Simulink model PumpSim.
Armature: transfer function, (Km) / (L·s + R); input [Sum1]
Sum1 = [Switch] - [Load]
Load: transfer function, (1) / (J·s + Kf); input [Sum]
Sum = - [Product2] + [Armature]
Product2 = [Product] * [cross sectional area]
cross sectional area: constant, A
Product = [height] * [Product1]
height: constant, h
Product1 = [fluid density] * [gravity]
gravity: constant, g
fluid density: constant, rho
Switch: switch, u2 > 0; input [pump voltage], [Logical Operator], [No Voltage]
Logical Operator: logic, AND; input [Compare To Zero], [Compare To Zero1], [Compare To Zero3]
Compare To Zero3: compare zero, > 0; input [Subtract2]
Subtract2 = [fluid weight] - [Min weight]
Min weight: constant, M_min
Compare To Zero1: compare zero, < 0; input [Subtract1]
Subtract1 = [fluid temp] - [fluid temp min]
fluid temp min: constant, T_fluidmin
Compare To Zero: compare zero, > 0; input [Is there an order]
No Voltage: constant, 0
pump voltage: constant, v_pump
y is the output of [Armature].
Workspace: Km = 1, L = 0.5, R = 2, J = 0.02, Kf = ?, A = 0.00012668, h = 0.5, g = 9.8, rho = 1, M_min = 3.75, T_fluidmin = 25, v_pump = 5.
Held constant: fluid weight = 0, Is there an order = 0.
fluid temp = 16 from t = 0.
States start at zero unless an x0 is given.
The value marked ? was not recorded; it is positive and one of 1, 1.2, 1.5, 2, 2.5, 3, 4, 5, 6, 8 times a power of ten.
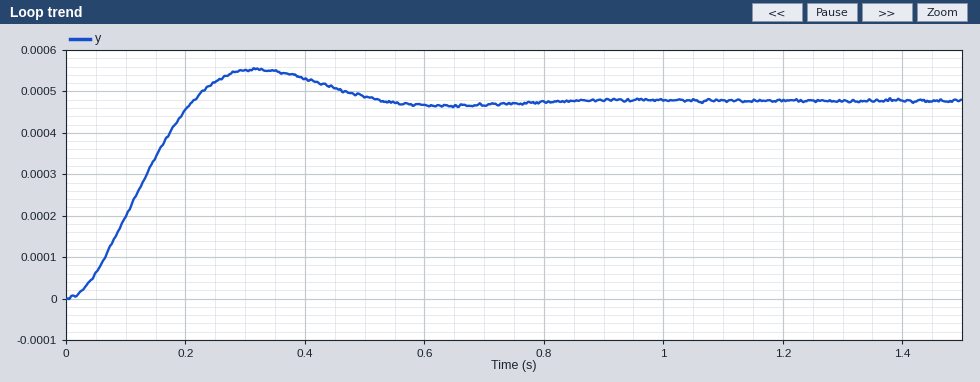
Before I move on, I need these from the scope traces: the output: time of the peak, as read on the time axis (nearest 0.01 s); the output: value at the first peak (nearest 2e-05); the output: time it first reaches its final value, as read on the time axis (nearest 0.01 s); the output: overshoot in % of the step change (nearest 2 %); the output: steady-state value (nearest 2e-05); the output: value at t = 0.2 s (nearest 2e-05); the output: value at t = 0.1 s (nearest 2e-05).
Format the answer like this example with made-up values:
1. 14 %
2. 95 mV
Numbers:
1. 0.32 s
2. 0.00056
3. 0.21 s
4. 16 %
5. 0.00048
6. 0.00046
7. 0.00020
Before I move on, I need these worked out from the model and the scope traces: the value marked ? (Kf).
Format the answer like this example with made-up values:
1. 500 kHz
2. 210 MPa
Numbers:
1. 0.15
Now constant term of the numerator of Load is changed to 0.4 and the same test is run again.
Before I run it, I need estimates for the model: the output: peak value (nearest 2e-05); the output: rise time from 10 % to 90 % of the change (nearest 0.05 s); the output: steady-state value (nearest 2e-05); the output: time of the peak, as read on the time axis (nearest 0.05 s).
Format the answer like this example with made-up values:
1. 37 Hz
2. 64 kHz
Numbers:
1. 0.00038
2. 0.25 s
3. 0.00036
4. 0.50 s
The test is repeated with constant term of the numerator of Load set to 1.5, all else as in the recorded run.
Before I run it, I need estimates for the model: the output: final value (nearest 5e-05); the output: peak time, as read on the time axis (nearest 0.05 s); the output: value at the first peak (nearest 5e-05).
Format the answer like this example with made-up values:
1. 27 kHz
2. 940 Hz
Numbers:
1. 0.00050
2. 0.25 s
3. 0.00065
